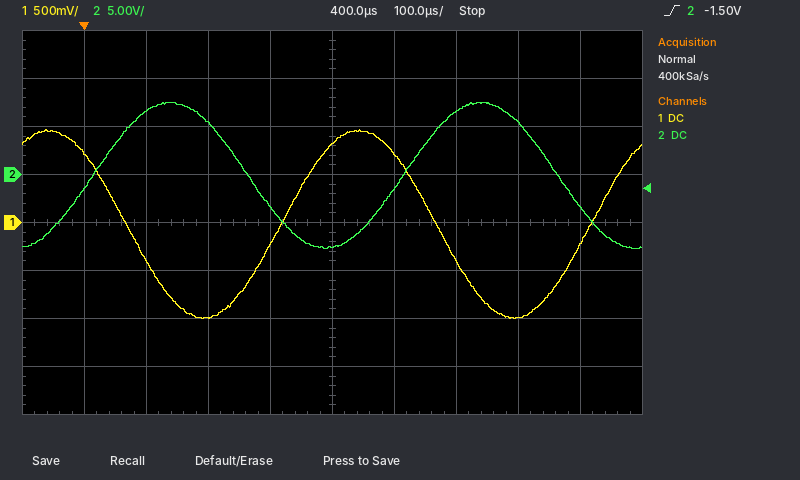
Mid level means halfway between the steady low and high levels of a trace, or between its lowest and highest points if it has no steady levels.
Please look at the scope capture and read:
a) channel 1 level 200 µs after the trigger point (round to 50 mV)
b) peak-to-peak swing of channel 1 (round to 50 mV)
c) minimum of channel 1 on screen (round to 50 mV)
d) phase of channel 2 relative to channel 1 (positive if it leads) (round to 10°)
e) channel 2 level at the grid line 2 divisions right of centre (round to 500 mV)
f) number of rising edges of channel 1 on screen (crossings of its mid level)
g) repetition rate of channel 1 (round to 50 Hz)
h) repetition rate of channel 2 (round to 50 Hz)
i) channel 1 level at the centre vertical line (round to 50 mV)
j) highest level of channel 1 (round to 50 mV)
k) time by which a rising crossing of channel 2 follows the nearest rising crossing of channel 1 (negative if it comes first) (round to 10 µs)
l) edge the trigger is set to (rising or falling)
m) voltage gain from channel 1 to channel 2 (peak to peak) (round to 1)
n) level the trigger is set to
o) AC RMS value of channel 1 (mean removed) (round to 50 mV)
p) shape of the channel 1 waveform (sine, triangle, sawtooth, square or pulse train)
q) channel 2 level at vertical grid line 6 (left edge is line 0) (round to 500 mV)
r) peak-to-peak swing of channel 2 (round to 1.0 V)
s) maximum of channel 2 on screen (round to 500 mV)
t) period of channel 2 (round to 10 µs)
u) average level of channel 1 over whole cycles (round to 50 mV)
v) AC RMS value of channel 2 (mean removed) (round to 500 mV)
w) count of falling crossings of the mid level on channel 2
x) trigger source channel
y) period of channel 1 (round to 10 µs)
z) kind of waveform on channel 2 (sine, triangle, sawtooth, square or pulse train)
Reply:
-1.00 V
1.95 V
-1.00 V
-140°
6.5 V
2
2.00 kHz
2.00 kHz
800 mV
950 mV
+200 µs
rising
8
-1.50 V
700 mV
sine
-1.5 V
15.0 V
7.5 V
500 µs
0 mV
5.5 V
2
channel 2
500 µs
sine
